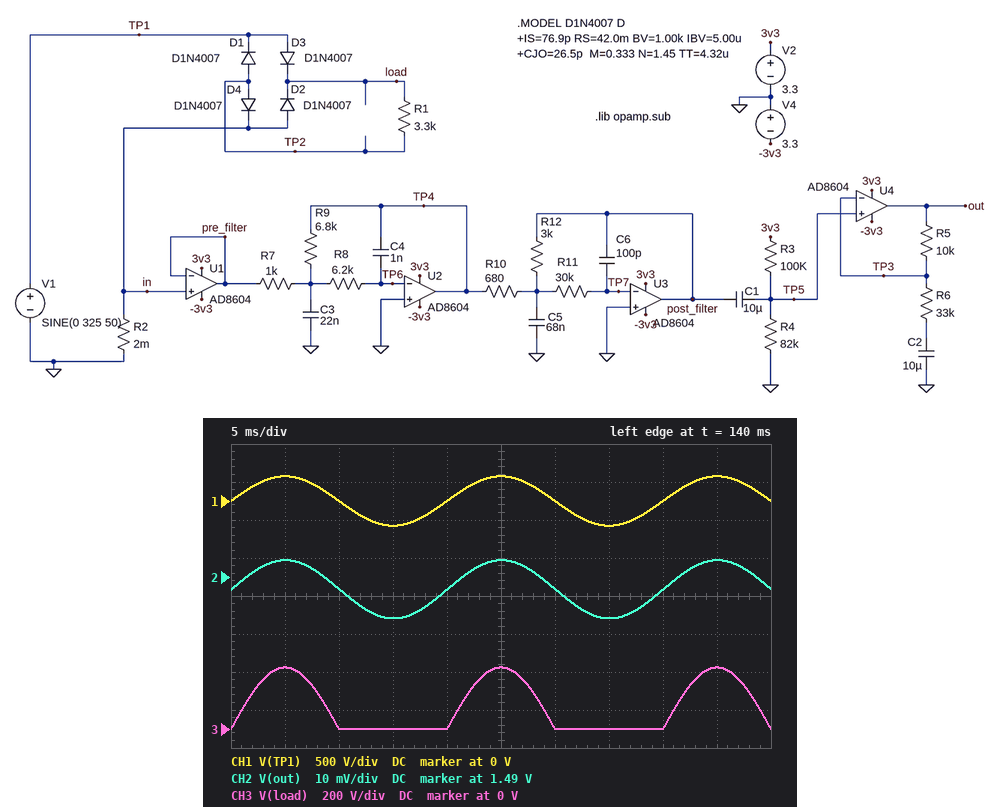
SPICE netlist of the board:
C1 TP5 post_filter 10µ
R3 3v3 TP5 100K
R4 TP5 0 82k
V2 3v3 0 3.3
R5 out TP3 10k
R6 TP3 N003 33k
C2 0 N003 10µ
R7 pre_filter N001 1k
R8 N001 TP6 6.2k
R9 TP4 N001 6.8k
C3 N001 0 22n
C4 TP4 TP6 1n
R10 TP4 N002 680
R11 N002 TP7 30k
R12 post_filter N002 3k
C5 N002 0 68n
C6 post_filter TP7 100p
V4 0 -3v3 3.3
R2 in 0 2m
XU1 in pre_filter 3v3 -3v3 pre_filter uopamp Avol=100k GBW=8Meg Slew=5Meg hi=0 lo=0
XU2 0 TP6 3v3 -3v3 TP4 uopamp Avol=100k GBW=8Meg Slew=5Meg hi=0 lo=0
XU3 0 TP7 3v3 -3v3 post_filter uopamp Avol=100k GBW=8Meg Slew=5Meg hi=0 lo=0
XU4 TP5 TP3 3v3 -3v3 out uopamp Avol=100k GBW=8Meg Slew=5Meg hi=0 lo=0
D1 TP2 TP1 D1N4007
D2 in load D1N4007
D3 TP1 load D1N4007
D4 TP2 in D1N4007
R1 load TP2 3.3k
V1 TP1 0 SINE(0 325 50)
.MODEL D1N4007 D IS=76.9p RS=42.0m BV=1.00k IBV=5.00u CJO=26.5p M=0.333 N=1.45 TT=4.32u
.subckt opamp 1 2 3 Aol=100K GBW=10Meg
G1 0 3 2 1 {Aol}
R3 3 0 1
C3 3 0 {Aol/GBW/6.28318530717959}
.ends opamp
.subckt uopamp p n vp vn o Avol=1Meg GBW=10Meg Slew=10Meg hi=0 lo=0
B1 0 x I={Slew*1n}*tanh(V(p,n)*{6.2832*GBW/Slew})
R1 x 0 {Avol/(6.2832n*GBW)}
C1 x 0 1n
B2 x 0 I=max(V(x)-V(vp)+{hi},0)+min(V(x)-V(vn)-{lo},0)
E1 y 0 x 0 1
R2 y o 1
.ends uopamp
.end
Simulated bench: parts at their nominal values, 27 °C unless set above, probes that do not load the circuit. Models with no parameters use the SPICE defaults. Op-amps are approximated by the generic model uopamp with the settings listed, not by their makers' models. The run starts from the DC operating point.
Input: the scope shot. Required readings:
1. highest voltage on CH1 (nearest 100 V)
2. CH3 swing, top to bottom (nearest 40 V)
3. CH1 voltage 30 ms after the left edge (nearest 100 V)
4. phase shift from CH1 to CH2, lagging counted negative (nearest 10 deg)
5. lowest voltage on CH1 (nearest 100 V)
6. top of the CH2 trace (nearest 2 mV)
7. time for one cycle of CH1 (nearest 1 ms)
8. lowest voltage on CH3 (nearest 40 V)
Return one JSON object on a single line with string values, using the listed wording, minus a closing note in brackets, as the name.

{"highest voltage on CH1": "300 V", "CH3 swing, top to bottom": "320 V", "CH1 voltage 30 ms after the left edge": "0 V", "phase shift from CH1 to CH2, lagging counted negative": "0 deg", "lowest voltage on CH1": "-300 V", "top of the CH2 trace": "1.494 V", "time for one cycle of CH1": "20 ms", "lowest voltage on CH3": "0 V"}
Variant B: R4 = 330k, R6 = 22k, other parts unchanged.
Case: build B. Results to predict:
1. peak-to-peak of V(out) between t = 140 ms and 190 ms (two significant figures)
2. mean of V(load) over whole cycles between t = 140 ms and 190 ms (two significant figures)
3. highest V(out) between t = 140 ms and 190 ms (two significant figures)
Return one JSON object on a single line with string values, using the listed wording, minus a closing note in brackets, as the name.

{"peak-to-peak of V(out) between t = 140 ms and 190 ms": "17 mV", "mean of V(load) over whole cycles between t = 140 ms and 190 ms": "100 V", "highest V(out) between t = 140 ms and 190 ms": "2.5 V"}
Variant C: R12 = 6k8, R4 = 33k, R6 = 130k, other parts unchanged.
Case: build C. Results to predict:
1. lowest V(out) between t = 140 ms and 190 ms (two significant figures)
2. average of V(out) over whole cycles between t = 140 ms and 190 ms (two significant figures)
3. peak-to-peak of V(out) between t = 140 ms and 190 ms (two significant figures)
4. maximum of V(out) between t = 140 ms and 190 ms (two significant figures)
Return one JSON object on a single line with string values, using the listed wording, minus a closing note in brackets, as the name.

{"lowest V(out) between t = 140 ms and 190 ms": "800 mV", "average of V(out) over whole cycles between t = 140 ms and 190 ms": "820 mV", "peak-to-peak of V(out) between t = 140 ms and 190 ms": "29 mV", "maximum of V(out) between t = 140 ms and 190 ms": "830 mV"}
